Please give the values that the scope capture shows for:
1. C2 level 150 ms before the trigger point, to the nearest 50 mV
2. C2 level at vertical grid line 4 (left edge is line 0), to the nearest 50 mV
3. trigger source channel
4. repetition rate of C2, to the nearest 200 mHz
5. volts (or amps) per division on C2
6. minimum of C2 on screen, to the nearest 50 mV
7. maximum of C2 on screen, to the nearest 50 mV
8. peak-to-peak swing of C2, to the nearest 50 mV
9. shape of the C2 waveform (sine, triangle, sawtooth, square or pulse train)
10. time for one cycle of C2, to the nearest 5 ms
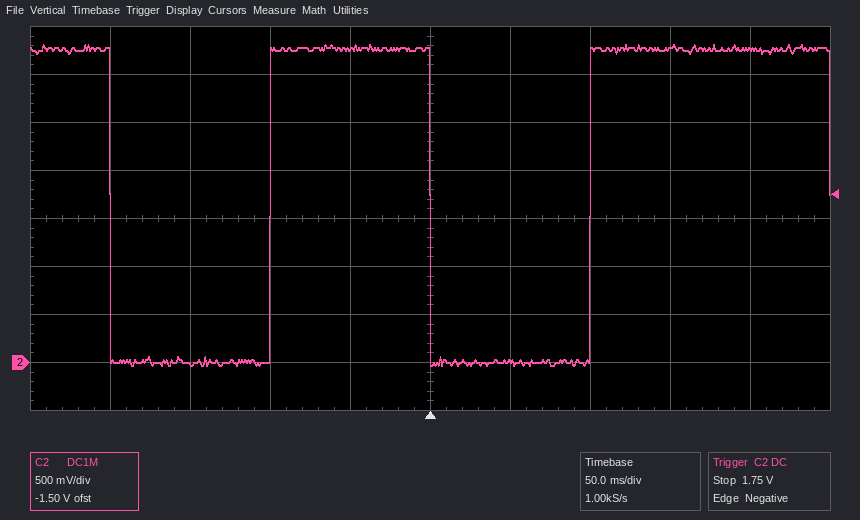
0 mV
3.25 V
C2
5.0 Hz
500 mV
-50 mV
3.30 V
3.35 V
square
200 ms
